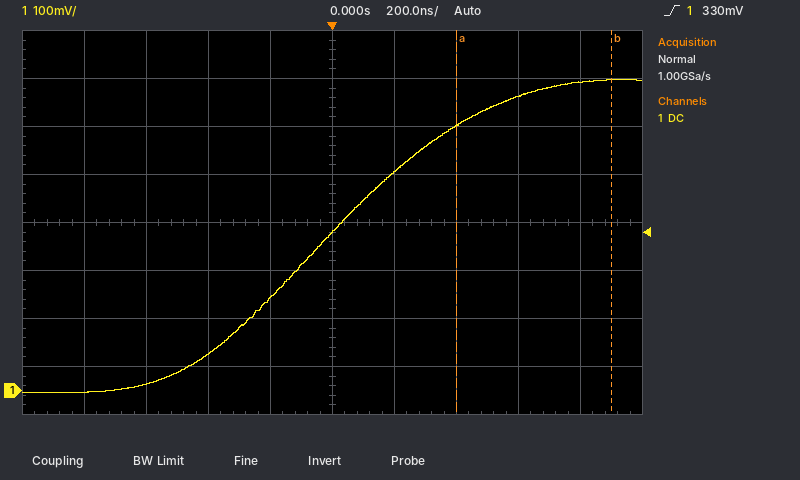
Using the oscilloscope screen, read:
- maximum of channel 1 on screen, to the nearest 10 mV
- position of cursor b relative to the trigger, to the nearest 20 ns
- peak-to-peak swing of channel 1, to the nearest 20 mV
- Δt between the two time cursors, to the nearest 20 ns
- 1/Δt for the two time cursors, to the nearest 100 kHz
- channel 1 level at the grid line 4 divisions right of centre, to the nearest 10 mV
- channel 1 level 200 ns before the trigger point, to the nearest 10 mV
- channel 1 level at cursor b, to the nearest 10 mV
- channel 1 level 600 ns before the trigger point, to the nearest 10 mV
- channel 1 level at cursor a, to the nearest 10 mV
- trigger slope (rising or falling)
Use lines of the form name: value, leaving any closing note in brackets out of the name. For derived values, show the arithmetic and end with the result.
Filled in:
maximum of channel 1 on screen, to the nearest 10 mV: 650 mV
position of cursor b relative to the trigger, to the nearest 20 ns: +900 ns
peak-to-peak swing of channel 1, to the nearest 20 mV: 660 mV
Δt between the two time cursors, to the nearest 20 ns: 500 ns
1/Δt for the two time cursors, to the nearest 100 kHz: 1 / 500 ns ≈ 2.0 MHz
channel 1 level at the grid line 4 divisions right of centre, to the nearest 10 mV: 640 mV
channel 1 level 200 ns before the trigger point, to the nearest 10 mV: 190 mV
channel 1 level at cursor b, to the nearest 10 mV: 650 mV
channel 1 level 600 ns before the trigger point, to the nearest 10 mV: 10 mV
channel 1 level at cursor a, to the nearest 10 mV: 550 mV
trigger slope: rising
